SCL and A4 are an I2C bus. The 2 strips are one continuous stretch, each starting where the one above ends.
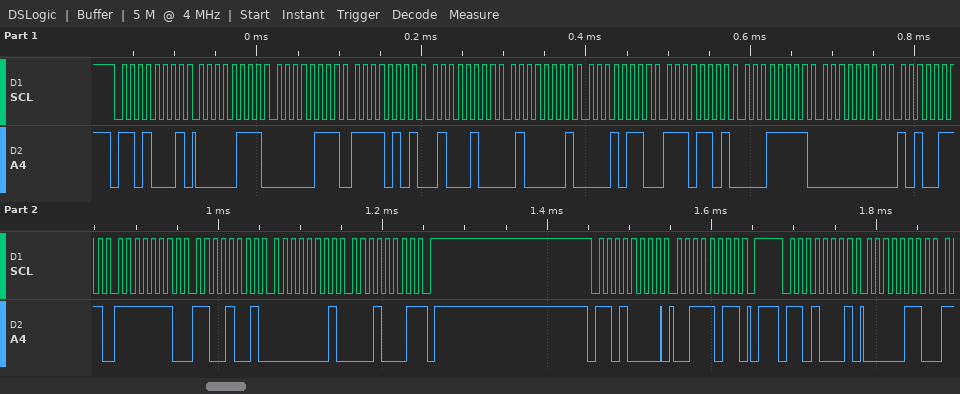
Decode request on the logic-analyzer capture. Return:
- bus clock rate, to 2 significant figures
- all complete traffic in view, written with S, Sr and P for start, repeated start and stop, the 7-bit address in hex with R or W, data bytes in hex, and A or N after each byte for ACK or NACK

100 kHz
S 68R A 07 A 07 A F5 A 44 A 41 A 16 A ED A 1F A 00 A A7 A FE A C9 A 01 A 11 N P S 68W A 3B A P S 68R A 06 A
